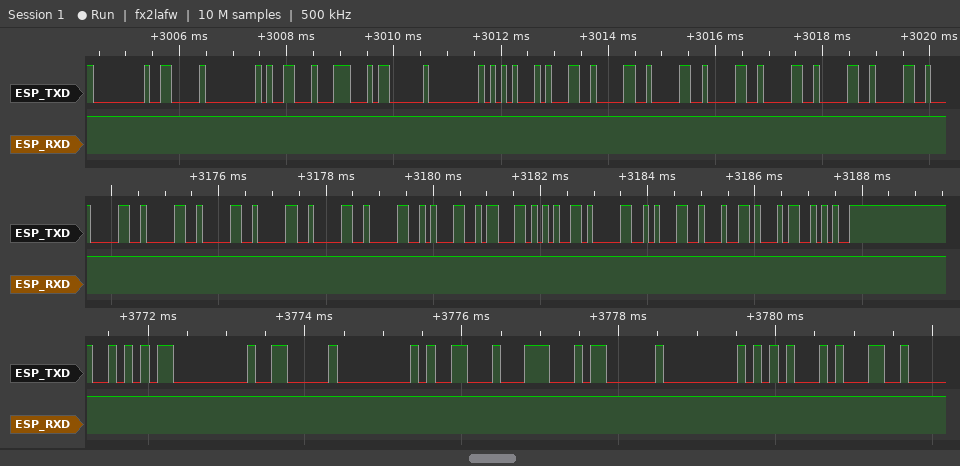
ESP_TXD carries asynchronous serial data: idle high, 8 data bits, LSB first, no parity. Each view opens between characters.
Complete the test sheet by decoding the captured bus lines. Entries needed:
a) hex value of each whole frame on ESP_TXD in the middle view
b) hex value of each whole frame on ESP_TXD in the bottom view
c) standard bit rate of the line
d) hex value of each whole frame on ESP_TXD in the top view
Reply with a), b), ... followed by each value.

a) 30, 30, 30, 30, 30, 30, 31, 63, 65, 30, 31, 64, 34, E5
b) AA, 00, 06, 00, 19, 1C, 03, 00, 15, 31
c) 9600 baud
d) 00, 06, 00, 19, 1C, 03, 00, 15, 31, 30, 30, 30, 30, 30, 30
